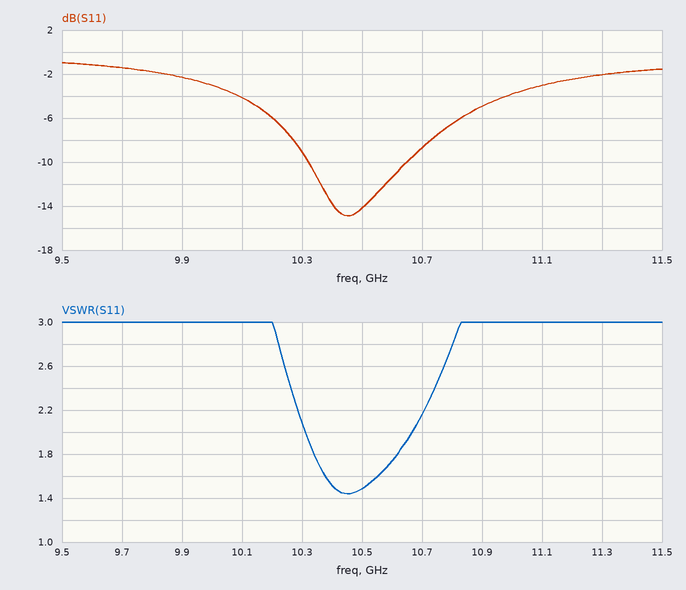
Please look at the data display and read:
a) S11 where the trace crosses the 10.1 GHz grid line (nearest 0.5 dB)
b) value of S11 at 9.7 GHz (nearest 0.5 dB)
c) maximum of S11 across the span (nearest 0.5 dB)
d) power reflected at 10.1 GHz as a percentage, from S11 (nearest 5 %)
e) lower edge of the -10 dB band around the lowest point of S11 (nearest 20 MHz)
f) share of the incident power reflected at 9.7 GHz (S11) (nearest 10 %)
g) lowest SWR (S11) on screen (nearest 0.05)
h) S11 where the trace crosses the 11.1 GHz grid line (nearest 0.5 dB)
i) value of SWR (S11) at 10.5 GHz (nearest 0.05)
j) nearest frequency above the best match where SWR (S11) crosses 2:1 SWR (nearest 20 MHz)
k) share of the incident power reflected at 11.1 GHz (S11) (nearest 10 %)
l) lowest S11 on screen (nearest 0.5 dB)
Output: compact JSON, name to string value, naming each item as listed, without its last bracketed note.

{"S11 where the trace crosses the 10.1 GHz grid line": "-4.0 dB", "value of S11 at 9.7 GHz": "-1.5 dB", "maximum of S11 across the span": "-1.0 dB", "power reflected at 10.1 GHz as a percentage, from S11": "40 %", "lower edge of the -10 dB band around the lowest point of S11": "10.32 GHz", "share of the incident power reflected at 9.7 GHz (S11)": "70 %", "lowest SWR (S11) on screen": "1.45", "S11 where the trace crosses the 11.1 GHz grid line": "-3.0 dB", "value of SWR (S11) at 10.5 GHz": "1.50", "nearest frequency above the best match where SWR (S11) crosses 2:1 SWR": "10.66 GHz", "share of the incident power reflected at 11.1 GHz (S11)": "50 %", "lowest S11 on screen": "-15.0 dB"}
